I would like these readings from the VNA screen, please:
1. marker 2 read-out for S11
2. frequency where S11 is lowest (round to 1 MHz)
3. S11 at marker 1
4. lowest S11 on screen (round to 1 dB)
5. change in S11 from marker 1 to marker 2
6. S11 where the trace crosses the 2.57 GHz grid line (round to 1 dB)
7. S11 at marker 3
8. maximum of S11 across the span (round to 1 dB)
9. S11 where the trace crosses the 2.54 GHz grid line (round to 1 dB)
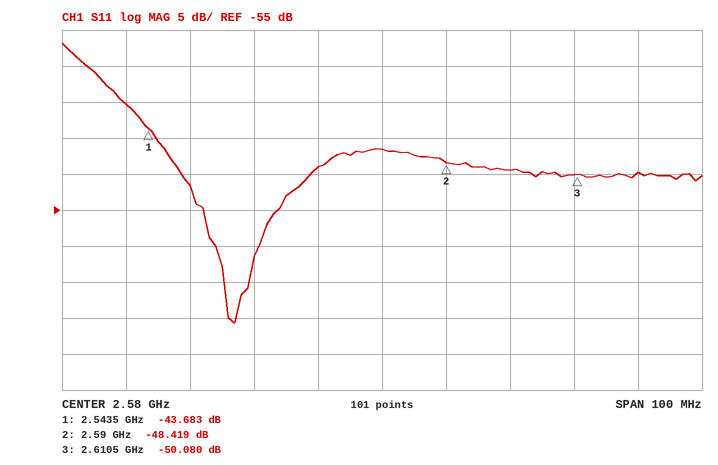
-48.419 dB
2.557 GHz
-43.683 dB
-71 dB
-4.736 dB
-49 dB
-50.080 dB
-32 dB
-40 dB
